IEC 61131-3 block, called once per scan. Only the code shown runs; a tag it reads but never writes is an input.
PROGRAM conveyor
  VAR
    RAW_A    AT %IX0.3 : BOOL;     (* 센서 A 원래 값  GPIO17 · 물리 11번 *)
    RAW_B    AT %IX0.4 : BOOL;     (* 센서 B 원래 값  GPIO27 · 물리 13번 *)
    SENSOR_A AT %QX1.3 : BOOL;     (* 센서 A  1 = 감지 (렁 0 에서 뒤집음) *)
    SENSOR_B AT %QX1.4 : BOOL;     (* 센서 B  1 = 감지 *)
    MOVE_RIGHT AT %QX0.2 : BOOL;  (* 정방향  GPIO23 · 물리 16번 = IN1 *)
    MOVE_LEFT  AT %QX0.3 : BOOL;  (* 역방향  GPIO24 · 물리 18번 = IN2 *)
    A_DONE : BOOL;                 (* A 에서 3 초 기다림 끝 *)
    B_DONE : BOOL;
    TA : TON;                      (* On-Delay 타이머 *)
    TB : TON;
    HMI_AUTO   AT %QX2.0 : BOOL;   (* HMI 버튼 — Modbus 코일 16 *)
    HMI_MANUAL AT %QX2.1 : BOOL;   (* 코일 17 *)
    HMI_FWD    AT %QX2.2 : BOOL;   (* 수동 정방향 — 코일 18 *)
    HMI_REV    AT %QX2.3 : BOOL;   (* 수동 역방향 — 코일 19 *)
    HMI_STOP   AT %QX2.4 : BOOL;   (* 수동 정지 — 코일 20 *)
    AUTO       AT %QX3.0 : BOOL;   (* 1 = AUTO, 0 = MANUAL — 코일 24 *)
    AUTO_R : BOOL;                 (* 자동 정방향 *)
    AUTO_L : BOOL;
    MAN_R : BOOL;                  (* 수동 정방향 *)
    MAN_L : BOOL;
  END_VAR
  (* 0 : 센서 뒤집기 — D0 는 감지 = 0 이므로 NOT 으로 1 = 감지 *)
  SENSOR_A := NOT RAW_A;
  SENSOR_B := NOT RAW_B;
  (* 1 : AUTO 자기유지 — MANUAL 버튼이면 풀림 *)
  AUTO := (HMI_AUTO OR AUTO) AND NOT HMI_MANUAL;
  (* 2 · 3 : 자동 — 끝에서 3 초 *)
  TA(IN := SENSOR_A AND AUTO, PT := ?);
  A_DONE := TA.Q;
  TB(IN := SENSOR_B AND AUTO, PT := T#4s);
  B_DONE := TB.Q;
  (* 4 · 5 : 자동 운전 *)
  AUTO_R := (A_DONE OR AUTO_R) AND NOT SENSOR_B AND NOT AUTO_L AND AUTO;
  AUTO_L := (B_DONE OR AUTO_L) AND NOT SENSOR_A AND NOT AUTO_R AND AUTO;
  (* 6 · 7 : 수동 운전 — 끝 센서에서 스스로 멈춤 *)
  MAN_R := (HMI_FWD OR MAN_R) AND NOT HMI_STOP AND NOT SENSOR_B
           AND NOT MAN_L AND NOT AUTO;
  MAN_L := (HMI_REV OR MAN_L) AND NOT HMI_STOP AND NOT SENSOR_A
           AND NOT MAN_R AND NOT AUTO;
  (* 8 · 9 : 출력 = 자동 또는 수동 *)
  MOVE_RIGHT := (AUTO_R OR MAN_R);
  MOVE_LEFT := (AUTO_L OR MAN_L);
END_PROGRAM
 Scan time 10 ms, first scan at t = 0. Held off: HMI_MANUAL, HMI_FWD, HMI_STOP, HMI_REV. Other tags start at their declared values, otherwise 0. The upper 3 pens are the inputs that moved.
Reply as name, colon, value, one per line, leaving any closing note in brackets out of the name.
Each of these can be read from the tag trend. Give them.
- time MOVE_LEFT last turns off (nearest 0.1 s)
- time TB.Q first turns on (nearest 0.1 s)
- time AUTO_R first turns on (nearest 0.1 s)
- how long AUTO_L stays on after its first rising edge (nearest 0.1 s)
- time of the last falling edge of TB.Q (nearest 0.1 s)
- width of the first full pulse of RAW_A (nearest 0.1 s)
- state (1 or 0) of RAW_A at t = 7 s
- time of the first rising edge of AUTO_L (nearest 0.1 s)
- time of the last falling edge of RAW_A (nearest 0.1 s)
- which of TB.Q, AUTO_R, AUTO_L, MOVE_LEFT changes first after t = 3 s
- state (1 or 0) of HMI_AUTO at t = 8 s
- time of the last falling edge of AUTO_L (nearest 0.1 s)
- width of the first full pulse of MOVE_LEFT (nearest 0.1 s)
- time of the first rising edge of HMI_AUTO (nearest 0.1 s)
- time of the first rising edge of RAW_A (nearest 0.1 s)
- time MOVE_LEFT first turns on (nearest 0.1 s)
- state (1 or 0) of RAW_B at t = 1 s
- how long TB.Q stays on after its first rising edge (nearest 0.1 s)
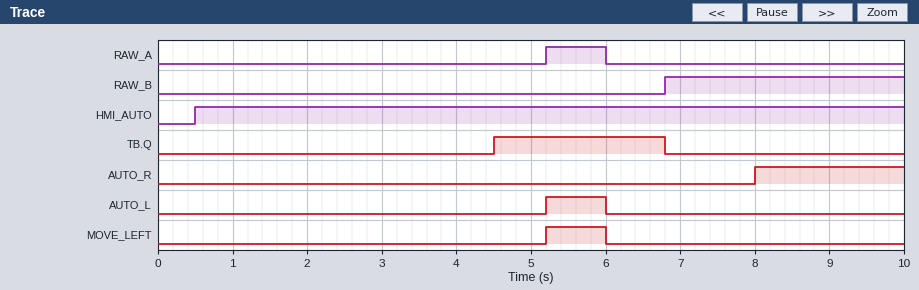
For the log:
time MOVE_LEFT last turns off: 6.0 s
time TB.Q first turns on: 4.5 s
time AUTO_R first turns on: 8.0 s
how long AUTO_L stays on after its first rising edge: 0.8 s
time of the last falling edge of TB.Q: 6.8 s
width of the first full pulse of RAW_A: 0.8 s
state (1 or 0) of RAW_A at t = 7 s: 0
time of the first rising edge of AUTO_L: 5.2 s
time of the last falling edge of RAW_A: 6.0 s
which of TB.Q, AUTO_R, AUTO_L, MOVE_LEFT changes first after t = 3 s: TB.Q
state (1 or 0) of HMI_AUTO at t = 8 s: 1
time of the last falling edge of AUTO_L: 6.0 s
width of the first full pulse of MOVE_LEFT: 0.8 s
time of the first rising edge of HMI_AUTO: 0.5 s
time of the first rising edge of RAW_A: 5.2 s
time MOVE_LEFT first turns on: 5.2 s
state (1 or 0) of RAW_B at t = 1 s: 0
how long TB.Q stays on after its first rising edge: 2.3 s
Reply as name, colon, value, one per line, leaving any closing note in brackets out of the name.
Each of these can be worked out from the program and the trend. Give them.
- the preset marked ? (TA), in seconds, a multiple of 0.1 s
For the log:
the preset marked ? (TA), in seconds, a multiple of 0.1 s: 2.0 s
